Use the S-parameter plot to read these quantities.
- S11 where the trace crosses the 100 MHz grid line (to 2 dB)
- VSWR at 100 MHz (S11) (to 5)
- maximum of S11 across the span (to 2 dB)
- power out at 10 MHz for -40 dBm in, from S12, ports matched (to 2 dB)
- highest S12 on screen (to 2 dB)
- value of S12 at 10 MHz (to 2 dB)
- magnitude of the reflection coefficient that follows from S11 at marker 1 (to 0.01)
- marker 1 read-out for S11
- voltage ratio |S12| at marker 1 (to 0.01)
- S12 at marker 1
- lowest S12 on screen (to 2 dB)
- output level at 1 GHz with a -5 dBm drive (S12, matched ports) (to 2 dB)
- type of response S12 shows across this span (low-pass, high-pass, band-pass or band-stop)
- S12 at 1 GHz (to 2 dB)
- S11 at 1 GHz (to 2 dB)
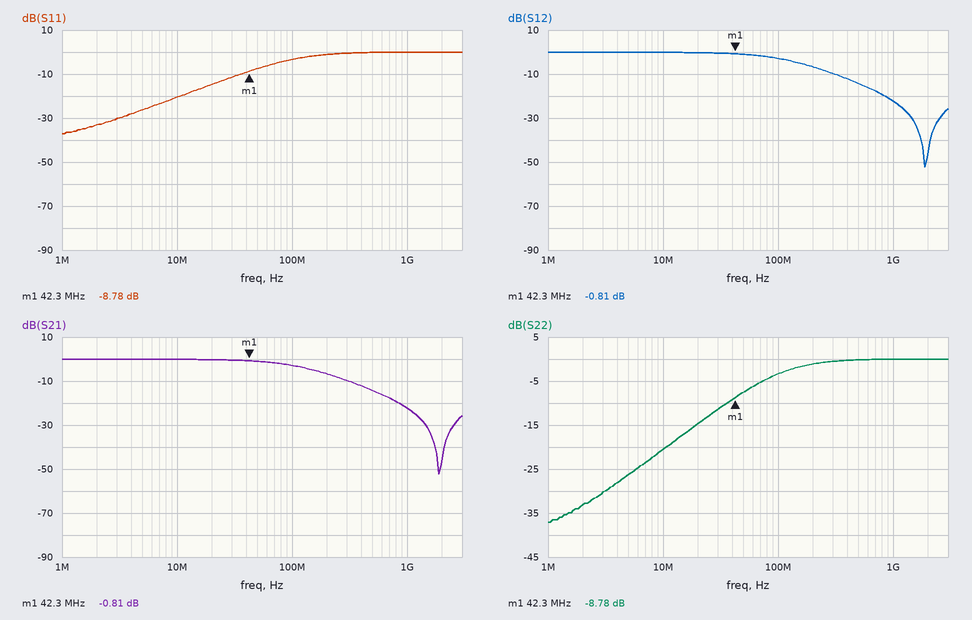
-4 dB
5
0 dB
-40 dBm
0 dB
0 dB
0.36
-8.78 dB
0.91
-0.81 dB
-52 dB
-28 dBm
low-pass
-22 dB
0 dB
